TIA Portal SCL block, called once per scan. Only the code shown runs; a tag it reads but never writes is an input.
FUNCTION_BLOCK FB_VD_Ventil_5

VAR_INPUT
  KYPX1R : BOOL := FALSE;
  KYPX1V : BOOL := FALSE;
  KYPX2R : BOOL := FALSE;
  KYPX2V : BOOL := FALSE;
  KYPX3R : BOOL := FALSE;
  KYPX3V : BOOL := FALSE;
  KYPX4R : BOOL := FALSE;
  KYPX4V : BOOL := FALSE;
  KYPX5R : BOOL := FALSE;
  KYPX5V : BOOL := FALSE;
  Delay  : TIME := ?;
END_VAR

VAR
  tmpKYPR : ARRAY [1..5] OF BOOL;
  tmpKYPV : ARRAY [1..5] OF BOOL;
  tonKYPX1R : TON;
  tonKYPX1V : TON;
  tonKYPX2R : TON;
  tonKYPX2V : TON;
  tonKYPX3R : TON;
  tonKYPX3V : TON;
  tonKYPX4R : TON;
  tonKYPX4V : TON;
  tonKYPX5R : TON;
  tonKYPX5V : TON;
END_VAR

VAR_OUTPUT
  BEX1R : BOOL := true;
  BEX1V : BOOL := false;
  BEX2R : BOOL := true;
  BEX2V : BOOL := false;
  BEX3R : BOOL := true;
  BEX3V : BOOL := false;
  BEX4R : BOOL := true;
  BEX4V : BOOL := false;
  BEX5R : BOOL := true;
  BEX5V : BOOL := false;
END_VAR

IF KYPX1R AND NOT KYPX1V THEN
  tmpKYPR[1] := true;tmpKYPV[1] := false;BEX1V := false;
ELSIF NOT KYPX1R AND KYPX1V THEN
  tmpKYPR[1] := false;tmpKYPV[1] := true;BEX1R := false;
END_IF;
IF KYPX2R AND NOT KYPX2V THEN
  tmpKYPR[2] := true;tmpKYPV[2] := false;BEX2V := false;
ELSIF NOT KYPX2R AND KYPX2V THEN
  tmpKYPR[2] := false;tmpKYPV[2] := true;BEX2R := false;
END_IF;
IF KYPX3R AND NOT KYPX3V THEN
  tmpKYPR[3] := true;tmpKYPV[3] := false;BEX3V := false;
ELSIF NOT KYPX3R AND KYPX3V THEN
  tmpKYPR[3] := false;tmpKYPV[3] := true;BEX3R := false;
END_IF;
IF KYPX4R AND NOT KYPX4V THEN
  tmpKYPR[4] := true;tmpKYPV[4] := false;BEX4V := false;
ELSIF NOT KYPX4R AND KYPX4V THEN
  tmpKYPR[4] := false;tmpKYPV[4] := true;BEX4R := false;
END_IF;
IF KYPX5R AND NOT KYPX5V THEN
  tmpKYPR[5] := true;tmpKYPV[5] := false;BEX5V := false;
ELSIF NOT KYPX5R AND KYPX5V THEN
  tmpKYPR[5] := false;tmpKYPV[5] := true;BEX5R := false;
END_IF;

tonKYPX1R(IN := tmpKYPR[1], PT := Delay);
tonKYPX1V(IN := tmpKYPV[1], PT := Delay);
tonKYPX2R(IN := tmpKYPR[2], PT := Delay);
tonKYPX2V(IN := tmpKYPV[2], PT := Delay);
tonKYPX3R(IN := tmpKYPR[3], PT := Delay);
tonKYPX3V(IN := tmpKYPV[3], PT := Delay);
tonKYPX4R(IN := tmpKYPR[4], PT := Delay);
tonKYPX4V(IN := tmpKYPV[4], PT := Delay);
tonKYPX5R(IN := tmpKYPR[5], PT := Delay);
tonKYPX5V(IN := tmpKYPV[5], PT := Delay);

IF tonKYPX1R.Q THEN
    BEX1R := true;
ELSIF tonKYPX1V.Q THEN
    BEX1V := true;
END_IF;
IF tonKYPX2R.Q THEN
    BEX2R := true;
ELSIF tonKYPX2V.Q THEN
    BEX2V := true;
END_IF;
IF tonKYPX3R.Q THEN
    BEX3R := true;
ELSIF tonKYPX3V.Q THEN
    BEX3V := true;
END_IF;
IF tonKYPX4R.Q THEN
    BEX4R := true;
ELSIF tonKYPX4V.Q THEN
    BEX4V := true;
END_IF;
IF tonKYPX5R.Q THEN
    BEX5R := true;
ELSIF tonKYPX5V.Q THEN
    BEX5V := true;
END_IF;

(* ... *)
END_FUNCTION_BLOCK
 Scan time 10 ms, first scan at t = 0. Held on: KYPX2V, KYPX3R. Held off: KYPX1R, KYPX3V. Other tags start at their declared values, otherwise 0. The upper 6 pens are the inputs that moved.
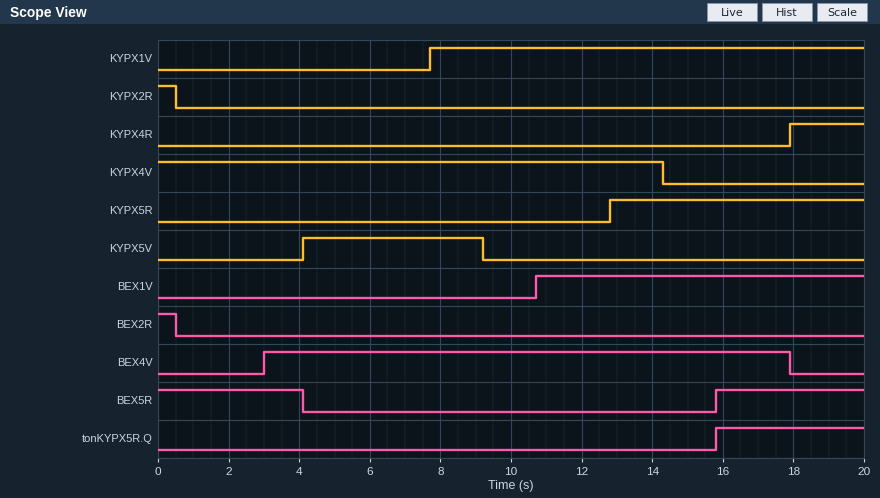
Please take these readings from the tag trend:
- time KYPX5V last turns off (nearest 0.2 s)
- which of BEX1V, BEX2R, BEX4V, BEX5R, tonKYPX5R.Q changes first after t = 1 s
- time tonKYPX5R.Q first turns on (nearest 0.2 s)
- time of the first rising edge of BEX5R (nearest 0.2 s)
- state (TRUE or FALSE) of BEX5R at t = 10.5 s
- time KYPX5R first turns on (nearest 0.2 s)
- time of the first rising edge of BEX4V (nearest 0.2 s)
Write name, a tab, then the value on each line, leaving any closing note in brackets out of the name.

time KYPX5V last turns off	9.2 s
which of BEX1V, BEX2R, BEX4V, BEX5R, tonKYPX5R.Q changes first after t = 1 s	BEX4V
time tonKYPX5R.Q first turns on	15.8 s
time of the first rising edge of BEX5R	15.8 s
state (TRUE or FALSE) of BEX5R at t = 10.5 s	FALSE
time KYPX5R first turns on	12.8 s
time of the first rising edge of BEX4V	3.0 s
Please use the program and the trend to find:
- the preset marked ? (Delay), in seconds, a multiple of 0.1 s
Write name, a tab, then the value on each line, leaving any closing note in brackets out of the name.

the preset marked ? (Delay), in seconds, a multiple of 0.1 s	3.0 s
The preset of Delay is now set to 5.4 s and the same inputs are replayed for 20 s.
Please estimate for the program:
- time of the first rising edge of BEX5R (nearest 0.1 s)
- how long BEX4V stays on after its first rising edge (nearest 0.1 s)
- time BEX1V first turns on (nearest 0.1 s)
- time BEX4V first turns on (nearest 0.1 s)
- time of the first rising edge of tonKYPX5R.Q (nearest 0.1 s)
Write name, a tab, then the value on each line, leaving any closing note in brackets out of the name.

time of the first rising edge of BEX5R	18.2 s
how long BEX4V stays on after its first rising edge	12.5 s
time BEX1V first turns on	13.1 s
time BEX4V first turns on	5.4 s
time of the first rising edge of tonKYPX5R.Q	18.2 s
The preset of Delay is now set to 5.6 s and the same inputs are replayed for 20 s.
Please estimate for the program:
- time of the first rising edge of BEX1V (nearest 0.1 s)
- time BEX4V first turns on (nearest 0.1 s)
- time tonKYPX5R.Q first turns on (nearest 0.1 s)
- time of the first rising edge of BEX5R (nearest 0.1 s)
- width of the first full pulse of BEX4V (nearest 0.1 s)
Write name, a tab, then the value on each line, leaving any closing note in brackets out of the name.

time of the first rising edge of BEX1V	13.3 s
time BEX4V first turns on	5.6 s
time tonKYPX5R.Q first turns on	18.4 s
time of the first rising edge of BEX5R	18.4 s
width of the first full pulse of BEX4V	12.3 s
